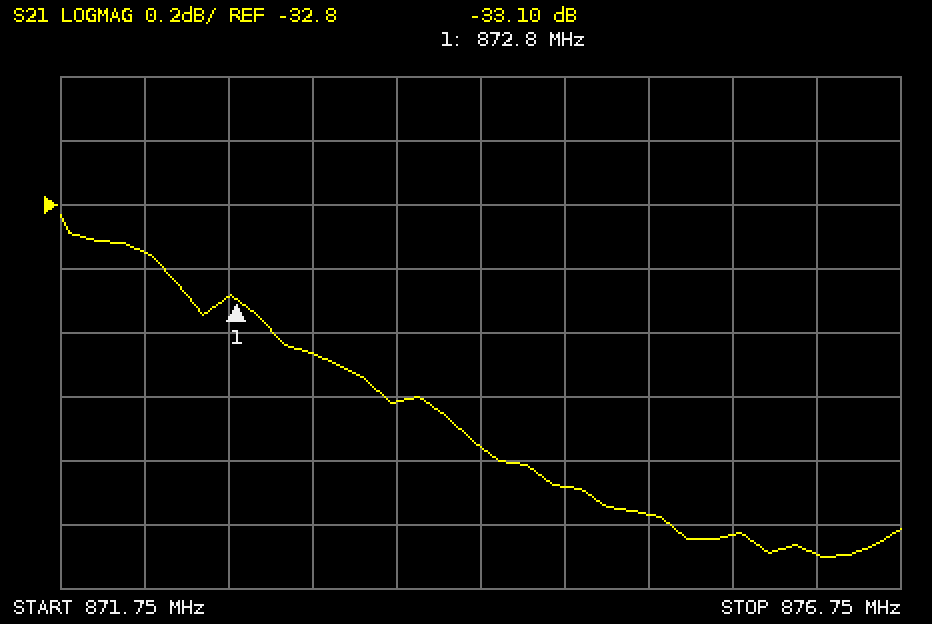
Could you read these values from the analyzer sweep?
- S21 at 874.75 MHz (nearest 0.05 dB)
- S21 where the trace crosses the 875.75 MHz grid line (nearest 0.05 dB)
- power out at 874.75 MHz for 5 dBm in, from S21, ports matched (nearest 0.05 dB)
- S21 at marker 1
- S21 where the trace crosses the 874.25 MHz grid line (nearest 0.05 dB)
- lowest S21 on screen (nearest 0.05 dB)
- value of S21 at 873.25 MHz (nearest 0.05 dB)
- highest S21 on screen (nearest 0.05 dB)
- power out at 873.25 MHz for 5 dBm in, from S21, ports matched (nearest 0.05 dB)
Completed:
-33.70 dB
-33.85 dB
-28.70 dBm
-33.10 dB
-33.55 dB
-33.90 dB
-33.25 dB
-32.85 dB
-28.25 dBm
